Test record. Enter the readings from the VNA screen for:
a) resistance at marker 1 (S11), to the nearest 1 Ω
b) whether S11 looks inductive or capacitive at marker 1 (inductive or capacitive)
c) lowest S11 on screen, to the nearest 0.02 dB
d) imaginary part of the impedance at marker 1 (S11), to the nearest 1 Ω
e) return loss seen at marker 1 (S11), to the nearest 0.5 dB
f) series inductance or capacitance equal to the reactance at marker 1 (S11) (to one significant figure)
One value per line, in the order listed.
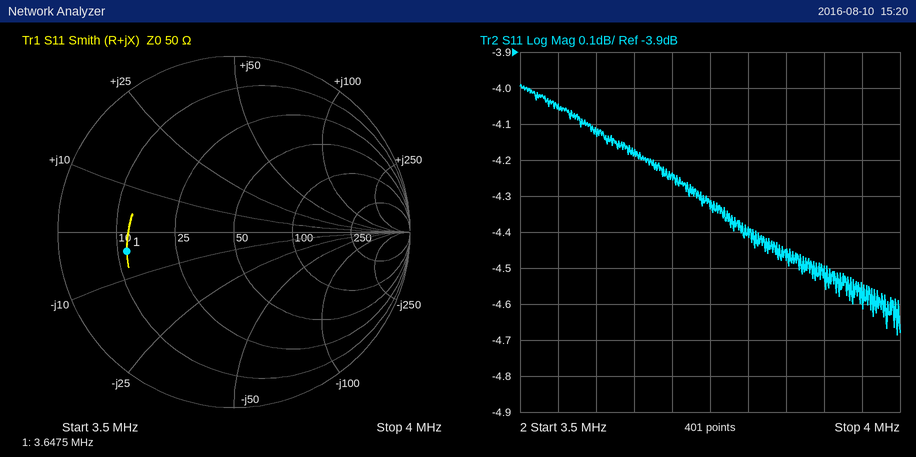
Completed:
12 Ω
capacitive
-4.68 dB
-4 Ω
4.0 dB
10 nF
